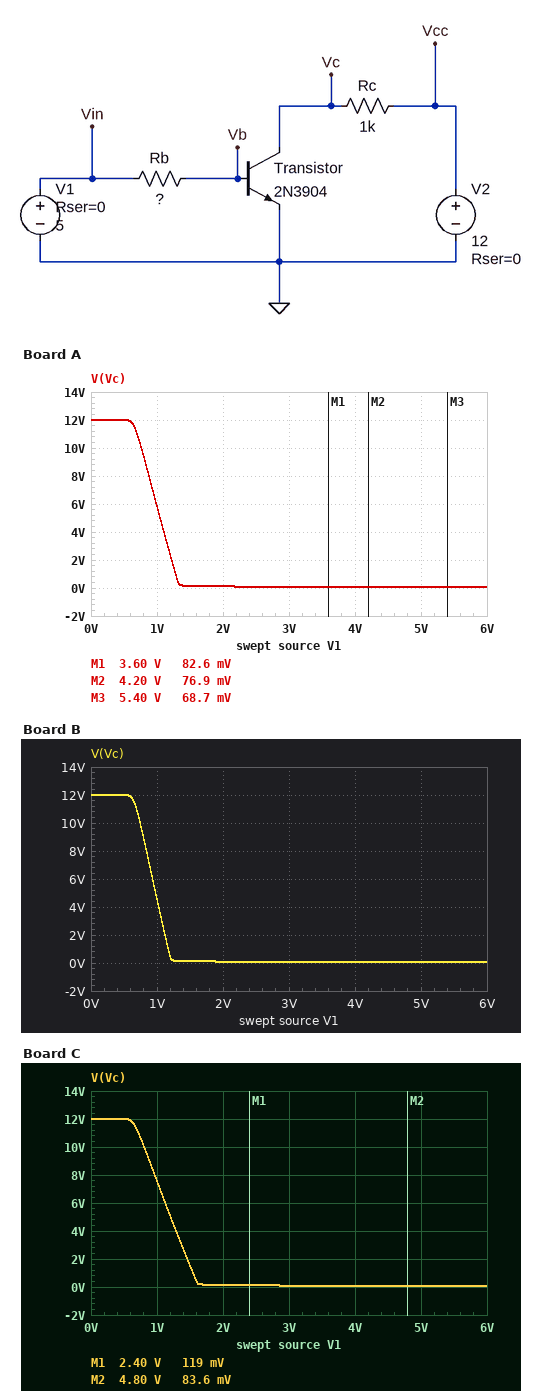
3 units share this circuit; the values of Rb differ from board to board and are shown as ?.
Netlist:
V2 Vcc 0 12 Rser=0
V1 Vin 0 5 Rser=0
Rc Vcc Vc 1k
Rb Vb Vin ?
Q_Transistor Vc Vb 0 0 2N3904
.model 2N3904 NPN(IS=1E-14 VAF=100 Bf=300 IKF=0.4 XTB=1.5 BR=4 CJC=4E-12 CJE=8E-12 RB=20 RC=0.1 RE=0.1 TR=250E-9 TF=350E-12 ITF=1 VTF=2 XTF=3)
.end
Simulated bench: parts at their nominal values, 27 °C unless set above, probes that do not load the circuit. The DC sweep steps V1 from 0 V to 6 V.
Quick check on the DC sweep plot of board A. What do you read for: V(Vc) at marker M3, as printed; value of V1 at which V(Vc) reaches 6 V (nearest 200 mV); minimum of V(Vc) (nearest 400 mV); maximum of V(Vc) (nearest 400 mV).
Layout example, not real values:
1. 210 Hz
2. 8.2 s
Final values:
1. 68.7 mV
2. 1.0 V
3. 0 V
4. 12.0 V
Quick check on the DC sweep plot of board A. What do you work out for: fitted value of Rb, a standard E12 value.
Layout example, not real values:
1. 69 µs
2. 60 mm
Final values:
1. 15 kΩ
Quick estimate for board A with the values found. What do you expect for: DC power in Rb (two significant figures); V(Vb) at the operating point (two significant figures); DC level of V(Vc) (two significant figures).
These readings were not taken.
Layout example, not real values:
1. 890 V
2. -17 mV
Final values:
1. 1.2 mW
2. 730 mV
3. 71 mV
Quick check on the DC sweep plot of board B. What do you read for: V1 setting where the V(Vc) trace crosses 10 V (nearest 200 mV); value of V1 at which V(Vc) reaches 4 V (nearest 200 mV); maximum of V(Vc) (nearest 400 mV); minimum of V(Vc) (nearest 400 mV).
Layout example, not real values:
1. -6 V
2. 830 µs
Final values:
1. 800 mV
2. 1.0 V
3. 12.0 V
4. 0 V
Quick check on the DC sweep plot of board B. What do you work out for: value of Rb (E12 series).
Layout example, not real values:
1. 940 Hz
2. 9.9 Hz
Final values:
1. 12 kΩ
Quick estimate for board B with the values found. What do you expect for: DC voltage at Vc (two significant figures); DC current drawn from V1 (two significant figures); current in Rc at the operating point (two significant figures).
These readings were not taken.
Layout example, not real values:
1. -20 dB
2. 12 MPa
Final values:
1. 65 mV
2. 360 µA
3. 12 mA
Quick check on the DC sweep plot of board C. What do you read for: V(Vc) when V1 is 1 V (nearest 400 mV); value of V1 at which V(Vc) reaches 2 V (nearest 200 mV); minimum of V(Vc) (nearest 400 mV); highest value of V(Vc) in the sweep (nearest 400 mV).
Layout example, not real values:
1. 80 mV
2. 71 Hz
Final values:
1. 7.6 V
2. 1.4 V
3. 0 V
4. 12.0 V
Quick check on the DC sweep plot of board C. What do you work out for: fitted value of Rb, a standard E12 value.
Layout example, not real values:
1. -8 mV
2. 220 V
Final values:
1. 22 kΩ
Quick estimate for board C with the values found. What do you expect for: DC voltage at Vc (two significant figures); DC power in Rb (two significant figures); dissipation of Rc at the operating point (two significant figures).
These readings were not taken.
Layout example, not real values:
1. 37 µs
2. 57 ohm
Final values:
1. 82 mV
2. 830 µW
3. 140 mW
